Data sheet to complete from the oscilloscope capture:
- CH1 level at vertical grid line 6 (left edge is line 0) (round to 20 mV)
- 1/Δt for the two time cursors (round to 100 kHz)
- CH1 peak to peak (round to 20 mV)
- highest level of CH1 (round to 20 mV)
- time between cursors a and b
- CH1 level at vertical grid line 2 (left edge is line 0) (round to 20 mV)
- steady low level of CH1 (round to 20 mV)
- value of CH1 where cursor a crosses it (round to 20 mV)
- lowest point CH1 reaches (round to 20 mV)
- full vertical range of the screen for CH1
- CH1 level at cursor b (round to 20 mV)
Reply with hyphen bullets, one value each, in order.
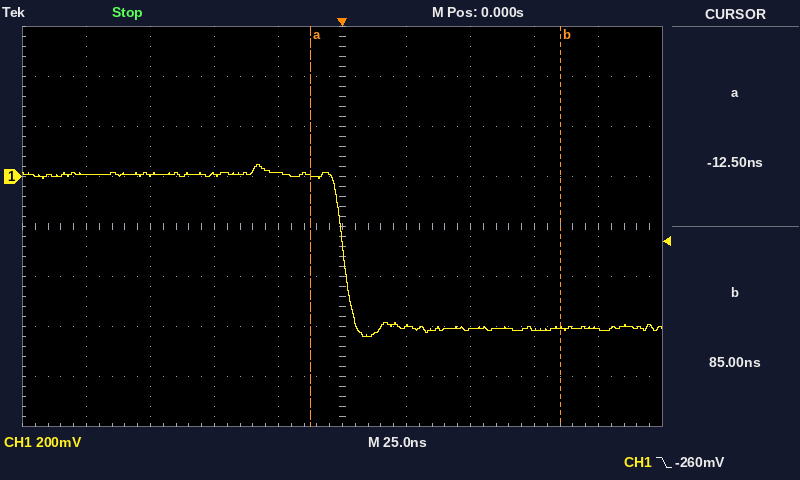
- -600 mV
- 10.3 MHz
- 680 mV
- 40 mV
- 97.5 ns
- 0 mV
- -600 mV
- 0 mV
- -640 mV
- 1.6 V
- -600 mV
